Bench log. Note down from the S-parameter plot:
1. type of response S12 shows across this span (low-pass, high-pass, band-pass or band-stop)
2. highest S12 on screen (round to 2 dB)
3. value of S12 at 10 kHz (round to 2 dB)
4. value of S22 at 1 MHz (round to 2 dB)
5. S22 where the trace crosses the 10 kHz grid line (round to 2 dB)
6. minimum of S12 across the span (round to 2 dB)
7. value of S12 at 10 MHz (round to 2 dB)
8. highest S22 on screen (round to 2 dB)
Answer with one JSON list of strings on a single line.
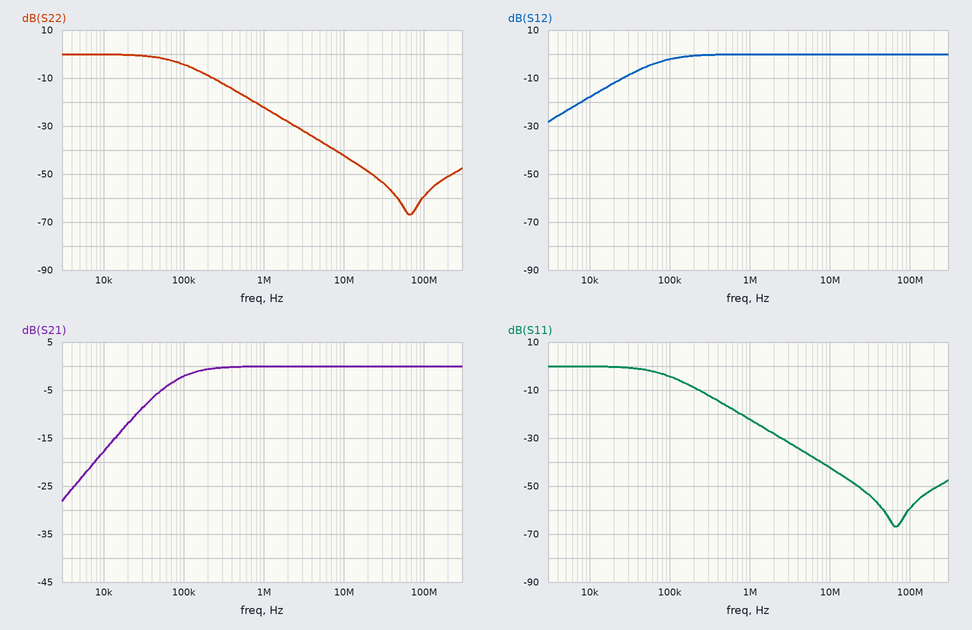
["high-pass", "0 dB", "-18 dB", "-22 dB", "0 dB", "-28 dB", "0 dB", "0 dB"]
